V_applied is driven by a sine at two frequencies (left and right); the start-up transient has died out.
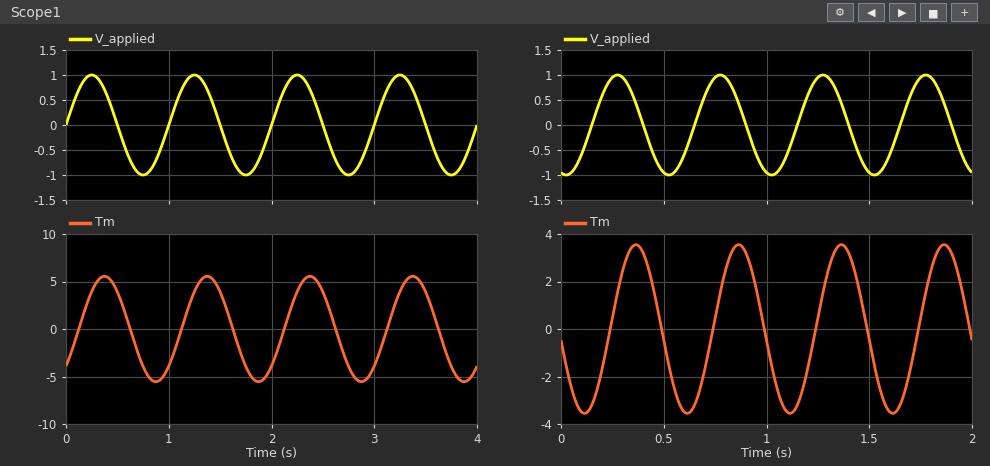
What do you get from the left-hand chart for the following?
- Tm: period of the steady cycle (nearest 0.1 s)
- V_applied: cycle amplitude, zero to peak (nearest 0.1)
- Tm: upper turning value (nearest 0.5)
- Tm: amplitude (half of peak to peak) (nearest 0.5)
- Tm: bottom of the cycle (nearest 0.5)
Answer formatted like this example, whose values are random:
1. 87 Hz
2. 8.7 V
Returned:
1. 1.0 s
2. 1.0
3. 5.5
4. 5.5
5. -5.5
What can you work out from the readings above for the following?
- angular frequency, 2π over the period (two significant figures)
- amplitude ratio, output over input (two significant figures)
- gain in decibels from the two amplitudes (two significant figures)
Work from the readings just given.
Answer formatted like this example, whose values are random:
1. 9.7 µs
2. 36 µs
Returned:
1. 6.3 rad/s
2. 5.5
3. 15 dB
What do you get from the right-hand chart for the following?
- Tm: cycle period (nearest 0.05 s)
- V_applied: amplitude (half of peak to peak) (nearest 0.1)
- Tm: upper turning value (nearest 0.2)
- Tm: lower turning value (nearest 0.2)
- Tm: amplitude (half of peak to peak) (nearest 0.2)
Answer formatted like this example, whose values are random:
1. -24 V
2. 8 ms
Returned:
1. 0.50 s
2. 1.0
3. 3.6
4. -3.6
5. 3.6
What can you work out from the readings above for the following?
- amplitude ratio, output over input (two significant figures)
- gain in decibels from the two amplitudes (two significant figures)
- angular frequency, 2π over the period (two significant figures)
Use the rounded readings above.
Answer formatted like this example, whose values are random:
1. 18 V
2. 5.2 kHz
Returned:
1. 3.6
2. 11 dB
3. 13 rad/s
